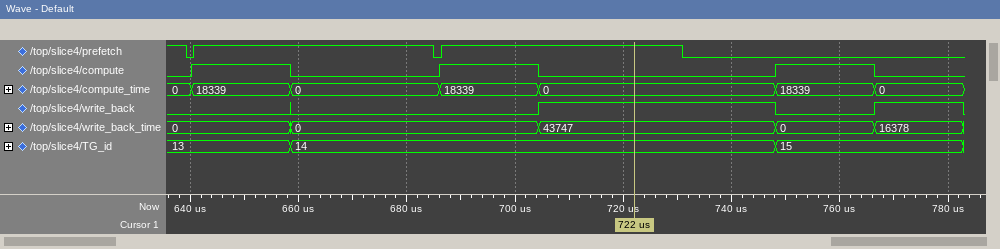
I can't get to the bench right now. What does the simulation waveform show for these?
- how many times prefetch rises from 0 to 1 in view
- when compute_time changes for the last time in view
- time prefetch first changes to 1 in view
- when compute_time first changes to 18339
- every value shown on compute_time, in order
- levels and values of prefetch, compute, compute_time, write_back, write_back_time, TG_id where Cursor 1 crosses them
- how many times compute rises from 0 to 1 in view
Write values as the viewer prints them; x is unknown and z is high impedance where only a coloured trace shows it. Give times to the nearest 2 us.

2
766 us
640 us
640 us
0, 18339, 0, 18339, 0, 18339, 0
prefetch=1, compute=0, compute_time=0, write_back=1, write_back_time=43747, TG_id=14
3
